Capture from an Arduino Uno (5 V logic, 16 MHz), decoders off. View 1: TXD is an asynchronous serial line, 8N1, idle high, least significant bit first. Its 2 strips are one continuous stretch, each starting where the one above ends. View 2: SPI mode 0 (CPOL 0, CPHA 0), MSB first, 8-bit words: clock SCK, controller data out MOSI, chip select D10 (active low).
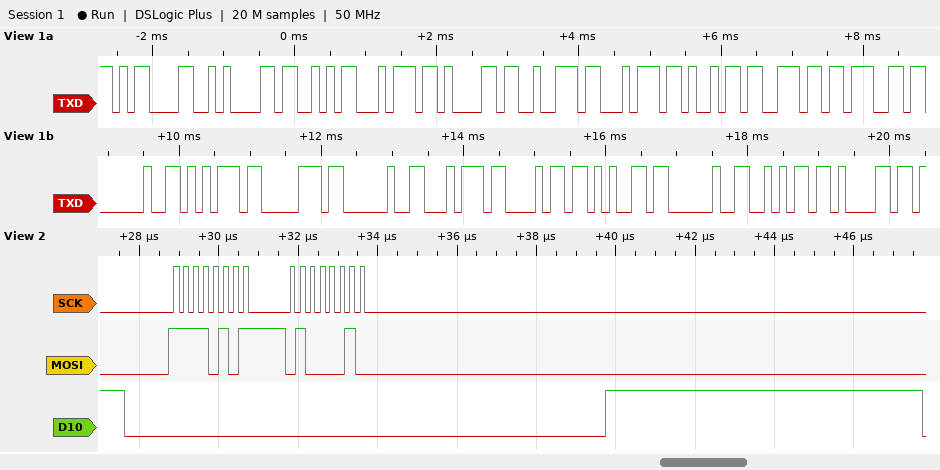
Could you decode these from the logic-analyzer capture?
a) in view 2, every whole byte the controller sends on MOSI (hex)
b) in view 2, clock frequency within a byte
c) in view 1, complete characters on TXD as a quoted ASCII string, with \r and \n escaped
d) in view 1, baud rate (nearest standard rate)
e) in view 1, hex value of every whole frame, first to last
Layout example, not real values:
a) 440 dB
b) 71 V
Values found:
a) F5 42
b) 4 MHz
c) "\r\nStarting up the ja"
d) 9600 baud
e) 0D 0A 53 74 61 72 74 69 6E 67 20 75 70 20 74 68 65 20 6A 61
